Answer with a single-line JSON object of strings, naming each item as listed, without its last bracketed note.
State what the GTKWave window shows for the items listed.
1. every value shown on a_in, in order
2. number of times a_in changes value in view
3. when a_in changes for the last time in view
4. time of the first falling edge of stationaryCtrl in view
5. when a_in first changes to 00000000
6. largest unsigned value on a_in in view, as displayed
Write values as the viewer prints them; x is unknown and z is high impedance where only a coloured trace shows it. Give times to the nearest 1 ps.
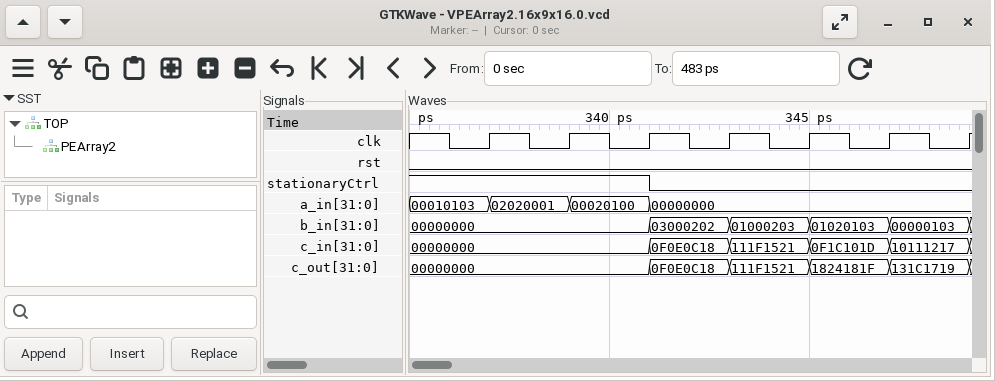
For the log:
{"every value shown on a_in, in order": "00010103, 02020001, 00020100, 00000000", "number of times a_in changes value in view": "3", "when a_in changes for the last time in view": "341 ps", "time of the first falling edge of stationaryCtrl in view": "341 ps", "when a_in first changes to 00000000": "341 ps", "largest unsigned value on a_in in view, as displayed": "02020001"}
